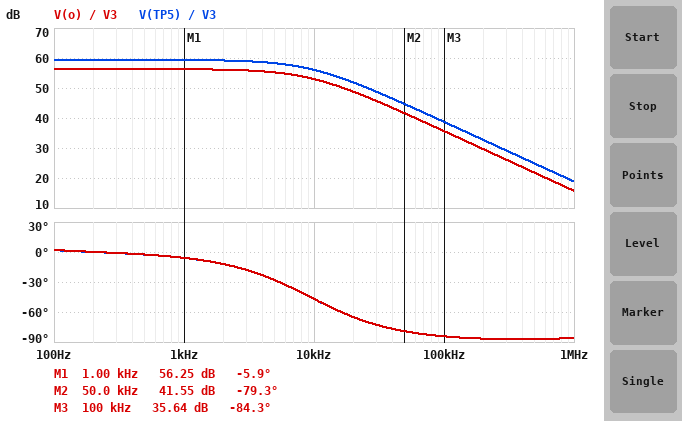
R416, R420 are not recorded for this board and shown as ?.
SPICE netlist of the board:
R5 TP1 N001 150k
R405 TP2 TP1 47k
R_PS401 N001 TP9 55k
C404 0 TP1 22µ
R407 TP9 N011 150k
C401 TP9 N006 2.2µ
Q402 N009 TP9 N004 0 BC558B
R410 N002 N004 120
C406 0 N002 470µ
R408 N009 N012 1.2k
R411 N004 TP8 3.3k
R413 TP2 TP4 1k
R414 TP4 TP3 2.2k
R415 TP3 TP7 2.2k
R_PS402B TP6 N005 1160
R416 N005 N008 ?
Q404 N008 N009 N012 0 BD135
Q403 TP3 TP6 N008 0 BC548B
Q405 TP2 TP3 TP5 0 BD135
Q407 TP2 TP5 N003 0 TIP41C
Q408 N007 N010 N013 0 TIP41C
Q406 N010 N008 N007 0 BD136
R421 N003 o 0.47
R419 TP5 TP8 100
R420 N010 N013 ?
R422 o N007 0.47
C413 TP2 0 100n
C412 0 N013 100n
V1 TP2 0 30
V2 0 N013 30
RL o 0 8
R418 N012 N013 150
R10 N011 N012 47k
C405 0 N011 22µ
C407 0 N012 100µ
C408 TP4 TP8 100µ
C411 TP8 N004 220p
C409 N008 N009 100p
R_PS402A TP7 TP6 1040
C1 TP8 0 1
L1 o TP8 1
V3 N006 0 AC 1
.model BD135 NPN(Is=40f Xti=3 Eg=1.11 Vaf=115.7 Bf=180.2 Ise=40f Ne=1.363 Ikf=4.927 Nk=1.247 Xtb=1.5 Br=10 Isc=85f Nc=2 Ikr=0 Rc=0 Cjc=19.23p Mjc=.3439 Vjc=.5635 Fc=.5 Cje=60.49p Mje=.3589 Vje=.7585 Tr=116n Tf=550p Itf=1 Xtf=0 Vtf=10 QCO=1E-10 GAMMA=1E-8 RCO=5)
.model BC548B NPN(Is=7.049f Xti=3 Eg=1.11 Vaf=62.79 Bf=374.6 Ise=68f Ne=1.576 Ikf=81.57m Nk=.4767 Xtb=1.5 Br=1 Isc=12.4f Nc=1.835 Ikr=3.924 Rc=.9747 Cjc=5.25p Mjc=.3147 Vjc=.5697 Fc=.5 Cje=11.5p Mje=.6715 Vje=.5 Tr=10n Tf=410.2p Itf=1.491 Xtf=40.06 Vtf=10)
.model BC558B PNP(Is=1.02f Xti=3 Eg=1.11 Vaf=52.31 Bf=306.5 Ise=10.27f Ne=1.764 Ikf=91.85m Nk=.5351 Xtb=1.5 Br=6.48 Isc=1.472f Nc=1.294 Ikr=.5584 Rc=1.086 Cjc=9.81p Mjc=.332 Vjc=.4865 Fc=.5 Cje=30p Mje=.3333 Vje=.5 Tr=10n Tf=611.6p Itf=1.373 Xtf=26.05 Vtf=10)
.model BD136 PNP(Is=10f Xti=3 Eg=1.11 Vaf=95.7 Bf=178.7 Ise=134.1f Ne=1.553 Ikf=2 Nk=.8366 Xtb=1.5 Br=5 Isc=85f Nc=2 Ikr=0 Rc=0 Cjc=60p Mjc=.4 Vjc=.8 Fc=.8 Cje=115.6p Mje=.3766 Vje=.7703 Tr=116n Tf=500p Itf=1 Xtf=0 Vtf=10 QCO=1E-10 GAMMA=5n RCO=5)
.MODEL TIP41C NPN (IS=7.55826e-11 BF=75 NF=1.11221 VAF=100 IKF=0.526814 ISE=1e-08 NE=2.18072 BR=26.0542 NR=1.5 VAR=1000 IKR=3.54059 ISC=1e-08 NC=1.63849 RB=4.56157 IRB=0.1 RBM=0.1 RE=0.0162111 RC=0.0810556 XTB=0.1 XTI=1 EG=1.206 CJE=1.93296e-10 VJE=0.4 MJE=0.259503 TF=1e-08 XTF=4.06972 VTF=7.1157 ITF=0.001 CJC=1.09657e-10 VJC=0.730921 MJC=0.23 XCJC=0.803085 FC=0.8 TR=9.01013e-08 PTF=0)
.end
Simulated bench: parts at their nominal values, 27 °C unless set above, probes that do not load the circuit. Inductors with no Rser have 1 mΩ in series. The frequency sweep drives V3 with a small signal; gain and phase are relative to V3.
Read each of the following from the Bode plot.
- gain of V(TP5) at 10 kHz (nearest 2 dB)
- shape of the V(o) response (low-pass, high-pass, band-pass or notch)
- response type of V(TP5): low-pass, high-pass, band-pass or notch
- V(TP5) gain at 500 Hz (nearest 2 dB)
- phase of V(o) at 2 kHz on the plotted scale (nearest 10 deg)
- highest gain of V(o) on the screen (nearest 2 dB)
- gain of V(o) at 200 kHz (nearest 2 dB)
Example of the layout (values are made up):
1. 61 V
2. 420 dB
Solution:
1. 56 dB
2. low-pass
3. low-pass
4. 60 dB
5. -10 deg
6. 56 dB
7. 30 dB
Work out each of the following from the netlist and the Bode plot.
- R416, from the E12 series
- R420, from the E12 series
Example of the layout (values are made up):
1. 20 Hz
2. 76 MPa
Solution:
1. 1.2 kΩ
2. 82 Ω
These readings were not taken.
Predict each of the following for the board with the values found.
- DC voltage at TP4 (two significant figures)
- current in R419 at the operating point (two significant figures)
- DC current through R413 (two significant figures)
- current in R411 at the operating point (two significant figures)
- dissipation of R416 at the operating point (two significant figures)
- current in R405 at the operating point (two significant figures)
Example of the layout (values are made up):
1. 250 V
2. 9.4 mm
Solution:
1. 21 V
2. 4.6 mA
3. 9.0 mA
4. 610 µA
5. 110 µW
6. 130 µA
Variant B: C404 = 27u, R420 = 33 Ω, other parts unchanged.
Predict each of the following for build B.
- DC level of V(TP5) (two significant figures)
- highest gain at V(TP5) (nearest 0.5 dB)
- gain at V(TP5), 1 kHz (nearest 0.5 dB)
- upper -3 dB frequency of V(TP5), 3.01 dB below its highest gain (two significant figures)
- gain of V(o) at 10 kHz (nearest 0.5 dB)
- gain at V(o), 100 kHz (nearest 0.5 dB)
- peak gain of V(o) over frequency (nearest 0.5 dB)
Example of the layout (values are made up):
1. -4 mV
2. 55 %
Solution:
1. 460 mV
2. 59.5 dB
3. 59.0 dB
4. 8.2 kHz
5. 52.0 dB
6. 35.0 dB
7. 56.0 dB
